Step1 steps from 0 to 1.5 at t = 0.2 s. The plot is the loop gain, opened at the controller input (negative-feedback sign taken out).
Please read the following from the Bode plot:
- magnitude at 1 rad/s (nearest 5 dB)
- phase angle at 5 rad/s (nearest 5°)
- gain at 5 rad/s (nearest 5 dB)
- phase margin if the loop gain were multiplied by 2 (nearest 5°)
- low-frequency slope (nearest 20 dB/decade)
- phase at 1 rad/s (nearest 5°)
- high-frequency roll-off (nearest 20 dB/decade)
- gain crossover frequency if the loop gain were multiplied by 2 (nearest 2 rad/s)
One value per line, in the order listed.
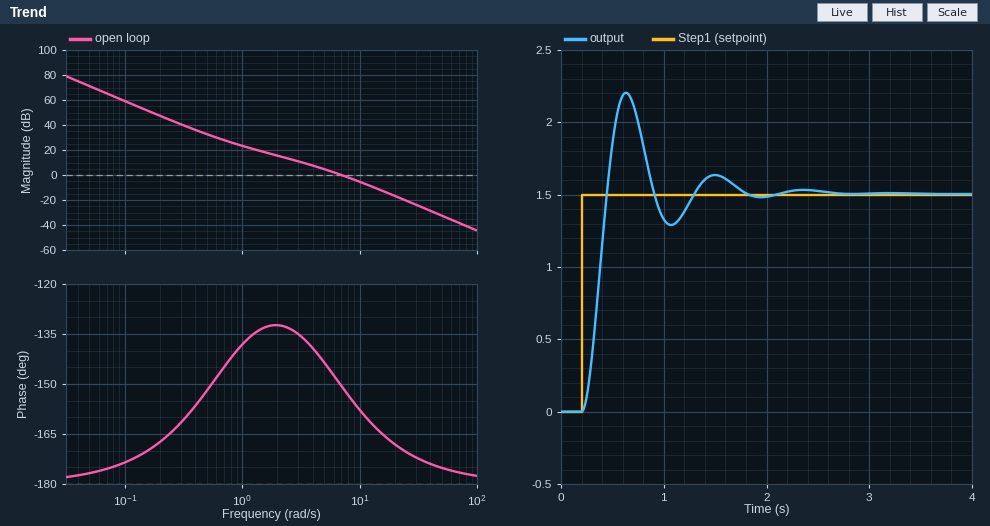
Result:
25 dB
-145°
5 dB
20°
-40 dB/decade
-140°
-40 dB/decade
10 rad/s
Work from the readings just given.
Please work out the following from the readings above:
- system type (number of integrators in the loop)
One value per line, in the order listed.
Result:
2
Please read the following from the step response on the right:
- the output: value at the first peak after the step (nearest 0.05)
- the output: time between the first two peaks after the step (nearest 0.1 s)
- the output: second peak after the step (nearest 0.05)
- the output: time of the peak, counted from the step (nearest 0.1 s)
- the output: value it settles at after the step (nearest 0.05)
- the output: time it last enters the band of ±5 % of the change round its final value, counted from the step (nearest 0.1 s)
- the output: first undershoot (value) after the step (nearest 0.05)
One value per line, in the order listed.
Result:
2.20
0.9 s
1.65
0.4 s
1.50
1.5 s
1.30
